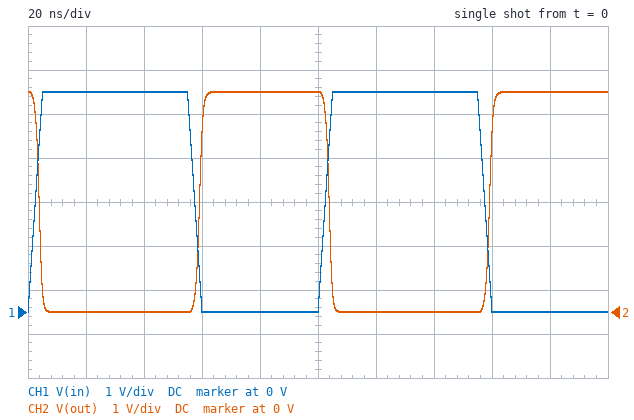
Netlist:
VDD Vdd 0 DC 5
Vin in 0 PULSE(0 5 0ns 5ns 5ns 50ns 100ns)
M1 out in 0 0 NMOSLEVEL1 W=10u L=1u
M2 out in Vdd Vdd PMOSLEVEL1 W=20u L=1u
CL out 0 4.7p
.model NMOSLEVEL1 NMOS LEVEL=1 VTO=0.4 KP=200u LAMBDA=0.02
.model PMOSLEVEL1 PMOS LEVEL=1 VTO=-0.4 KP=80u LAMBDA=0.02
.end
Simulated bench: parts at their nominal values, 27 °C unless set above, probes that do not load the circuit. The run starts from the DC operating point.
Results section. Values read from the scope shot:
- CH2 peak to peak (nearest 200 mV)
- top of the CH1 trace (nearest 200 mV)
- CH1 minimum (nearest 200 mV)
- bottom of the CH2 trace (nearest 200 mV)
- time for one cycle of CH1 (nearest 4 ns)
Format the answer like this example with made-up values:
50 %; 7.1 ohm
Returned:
5.0 V; 5.0 V; 0 V; 0 V; 100 ns
